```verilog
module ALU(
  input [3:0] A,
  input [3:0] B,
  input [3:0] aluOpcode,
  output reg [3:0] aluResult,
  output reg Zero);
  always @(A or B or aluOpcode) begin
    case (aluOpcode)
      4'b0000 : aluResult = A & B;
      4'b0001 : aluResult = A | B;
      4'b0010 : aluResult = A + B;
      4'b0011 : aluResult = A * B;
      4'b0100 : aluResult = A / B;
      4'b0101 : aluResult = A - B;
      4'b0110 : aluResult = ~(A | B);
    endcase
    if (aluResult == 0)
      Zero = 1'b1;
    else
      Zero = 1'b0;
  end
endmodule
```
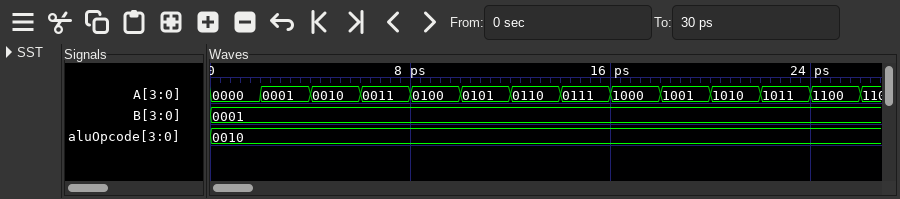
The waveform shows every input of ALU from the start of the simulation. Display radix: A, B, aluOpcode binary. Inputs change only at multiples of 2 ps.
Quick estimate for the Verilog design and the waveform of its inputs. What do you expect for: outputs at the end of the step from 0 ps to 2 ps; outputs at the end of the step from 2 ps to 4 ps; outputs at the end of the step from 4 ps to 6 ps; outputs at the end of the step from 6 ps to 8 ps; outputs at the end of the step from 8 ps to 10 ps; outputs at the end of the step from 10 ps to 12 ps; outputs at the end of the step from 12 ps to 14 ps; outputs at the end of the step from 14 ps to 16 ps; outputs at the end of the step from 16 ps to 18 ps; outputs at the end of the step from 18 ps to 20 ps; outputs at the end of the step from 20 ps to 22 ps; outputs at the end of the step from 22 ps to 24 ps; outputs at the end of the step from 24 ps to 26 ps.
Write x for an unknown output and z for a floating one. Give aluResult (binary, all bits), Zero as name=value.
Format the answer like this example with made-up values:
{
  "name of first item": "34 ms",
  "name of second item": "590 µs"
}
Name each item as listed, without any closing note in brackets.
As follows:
{
  "outputs at the end of the step from 0 ps to 2 ps": "aluResult=0001, Zero=0",
  "outputs at the end of the step from 2 ps to 4 ps": "aluResult=0010, Zero=0",
  "outputs at the end of the step from 4 ps to 6 ps": "aluResult=0011, Zero=0",
  "outputs at the end of the step from 6 ps to 8 ps": "aluResult=0100, Zero=0",
  "outputs at the end of the step from 8 ps to 10 ps": "aluResult=0101, Zero=0",
  "outputs at the end of the step from 10 ps to 12 ps": "aluResult=0110, Zero=0",
  "outputs at the end of the step from 12 ps to 14 ps": "aluResult=0111, Zero=0",
  "outputs at the end of the step from 14 ps to 16 ps": "aluResult=1000, Zero=0",
  "outputs at the end of the step from 16 ps to 18 ps": "aluResult=1001, Zero=0",
  "outputs at the end of the step from 18 ps to 20 ps": "aluResult=1010, Zero=0",
  "outputs at the end of the step from 20 ps to 22 ps": "aluResult=1011, Zero=0",
  "outputs at the end of the step from 22 ps to 24 ps": "aluResult=1100, Zero=0",
  "outputs at the end of the step from 24 ps to 26 ps": "aluResult=1101, Zero=0"
}
